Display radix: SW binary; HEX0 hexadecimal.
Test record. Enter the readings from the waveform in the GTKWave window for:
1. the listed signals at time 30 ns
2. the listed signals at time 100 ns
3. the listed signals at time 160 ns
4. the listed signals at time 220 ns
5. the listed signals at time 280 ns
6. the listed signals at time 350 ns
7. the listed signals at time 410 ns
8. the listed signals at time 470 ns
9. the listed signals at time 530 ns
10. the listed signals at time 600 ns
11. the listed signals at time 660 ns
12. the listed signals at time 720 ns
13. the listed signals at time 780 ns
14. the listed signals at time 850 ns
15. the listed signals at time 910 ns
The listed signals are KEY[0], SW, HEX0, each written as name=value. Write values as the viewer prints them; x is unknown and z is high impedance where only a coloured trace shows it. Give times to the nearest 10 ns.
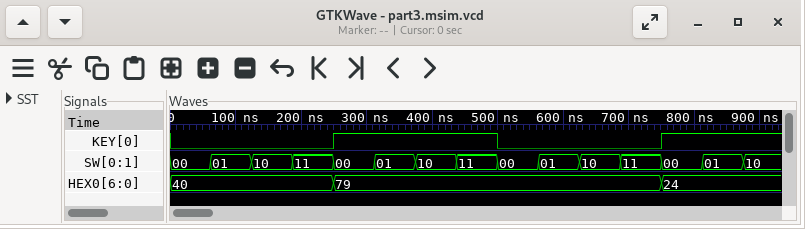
KEY[0]=0, SW=00, HEX0=40
KEY[0]=0, SW=01, HEX0=40
KEY[0]=0, SW=10, HEX0=40
KEY[0]=0, SW=11, HEX0=40
KEY[0]=1, SW=00, HEX0=79
KEY[0]=1, SW=01, HEX0=79
KEY[0]=1, SW=10, HEX0=79
KEY[0]=1, SW=11, HEX0=79
KEY[0]=0, SW=00, HEX0=79
KEY[0]=0, SW=01, HEX0=79
KEY[0]=0, SW=10, HEX0=79
KEY[0]=0, SW=11, HEX0=79
KEY[0]=1, SW=00, HEX0=24
KEY[0]=1, SW=01, HEX0=24
KEY[0]=1, SW=10, HEX0=24
